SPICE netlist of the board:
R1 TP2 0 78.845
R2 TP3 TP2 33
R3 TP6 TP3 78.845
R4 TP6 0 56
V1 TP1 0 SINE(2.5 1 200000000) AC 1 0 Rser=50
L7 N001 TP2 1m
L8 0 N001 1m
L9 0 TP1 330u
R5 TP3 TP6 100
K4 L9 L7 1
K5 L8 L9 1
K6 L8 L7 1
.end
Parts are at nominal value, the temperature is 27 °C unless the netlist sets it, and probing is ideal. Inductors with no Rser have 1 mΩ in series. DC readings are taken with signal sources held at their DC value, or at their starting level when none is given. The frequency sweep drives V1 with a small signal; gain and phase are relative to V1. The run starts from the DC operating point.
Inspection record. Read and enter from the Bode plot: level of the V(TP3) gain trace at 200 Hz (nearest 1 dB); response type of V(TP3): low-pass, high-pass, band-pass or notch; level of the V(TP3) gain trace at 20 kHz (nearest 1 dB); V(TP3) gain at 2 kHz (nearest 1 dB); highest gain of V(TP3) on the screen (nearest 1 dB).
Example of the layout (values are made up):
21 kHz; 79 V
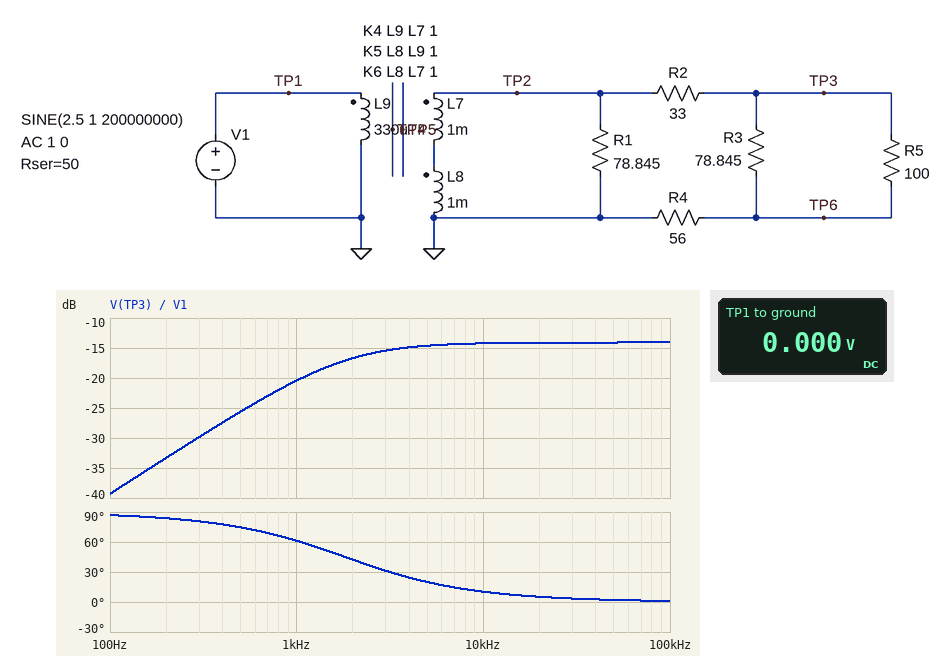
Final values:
-33 dB; high-pass; -14 dB; -17 dB; -14 dB
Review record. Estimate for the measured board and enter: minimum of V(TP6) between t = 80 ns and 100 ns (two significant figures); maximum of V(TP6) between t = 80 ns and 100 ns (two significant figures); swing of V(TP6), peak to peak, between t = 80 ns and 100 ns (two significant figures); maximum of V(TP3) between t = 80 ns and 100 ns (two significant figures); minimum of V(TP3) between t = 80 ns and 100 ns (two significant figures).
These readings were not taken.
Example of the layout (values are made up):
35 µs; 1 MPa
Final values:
-110 mV; 110 mV; 220 mV; 200 mV; -200 mV
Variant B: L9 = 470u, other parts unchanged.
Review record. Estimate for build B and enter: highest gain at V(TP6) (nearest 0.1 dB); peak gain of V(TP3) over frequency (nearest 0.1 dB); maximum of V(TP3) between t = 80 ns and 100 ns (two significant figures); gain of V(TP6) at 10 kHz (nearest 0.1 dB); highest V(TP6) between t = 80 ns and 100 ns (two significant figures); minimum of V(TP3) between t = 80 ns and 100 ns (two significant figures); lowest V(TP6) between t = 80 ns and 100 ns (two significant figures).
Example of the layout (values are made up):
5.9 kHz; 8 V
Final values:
-17.9 dB; -12.8 dB; 230 mV; -18.0 dB; 130 mV; -230 mV; -130 mV
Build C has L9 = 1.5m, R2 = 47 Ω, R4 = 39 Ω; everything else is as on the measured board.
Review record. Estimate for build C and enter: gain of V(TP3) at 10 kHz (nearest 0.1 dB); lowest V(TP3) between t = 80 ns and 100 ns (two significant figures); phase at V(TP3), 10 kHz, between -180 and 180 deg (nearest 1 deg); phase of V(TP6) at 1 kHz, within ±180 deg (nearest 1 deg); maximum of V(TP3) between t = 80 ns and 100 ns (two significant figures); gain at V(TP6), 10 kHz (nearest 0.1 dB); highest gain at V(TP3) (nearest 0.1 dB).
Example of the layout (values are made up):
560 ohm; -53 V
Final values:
-11.1 dB; -280 mV; 8 deg; 55 deg; 280 mV; -17.7 dB; -11.0 dB
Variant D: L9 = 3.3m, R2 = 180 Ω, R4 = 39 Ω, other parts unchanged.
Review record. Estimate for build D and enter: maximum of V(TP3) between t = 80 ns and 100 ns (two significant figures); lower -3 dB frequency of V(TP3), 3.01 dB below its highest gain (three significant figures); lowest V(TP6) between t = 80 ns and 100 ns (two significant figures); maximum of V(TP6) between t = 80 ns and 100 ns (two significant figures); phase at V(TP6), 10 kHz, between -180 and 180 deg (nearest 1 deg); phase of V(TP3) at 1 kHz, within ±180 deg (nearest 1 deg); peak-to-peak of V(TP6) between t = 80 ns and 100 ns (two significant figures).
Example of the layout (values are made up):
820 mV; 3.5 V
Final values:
170 mV; 1.21 kHz; -82 mV; 82 mV; 7 deg; 50 deg; 160 mV
